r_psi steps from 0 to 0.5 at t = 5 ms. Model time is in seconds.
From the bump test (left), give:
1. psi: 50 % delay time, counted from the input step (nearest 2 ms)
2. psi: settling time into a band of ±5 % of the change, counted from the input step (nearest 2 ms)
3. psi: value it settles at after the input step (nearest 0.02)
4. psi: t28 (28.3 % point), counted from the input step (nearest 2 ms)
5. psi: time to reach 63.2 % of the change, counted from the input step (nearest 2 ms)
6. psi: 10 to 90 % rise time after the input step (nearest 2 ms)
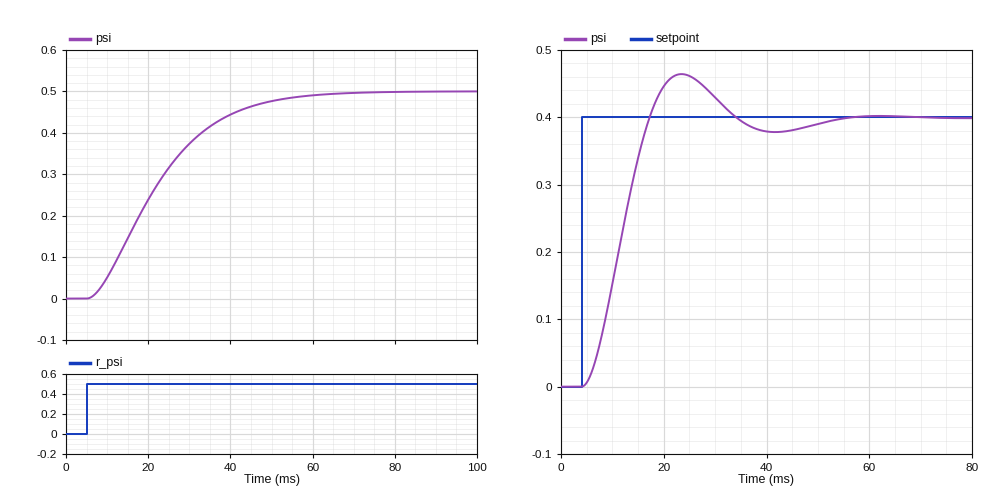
16 ms
44 ms
0.50
10 ms
20 ms
32 ms
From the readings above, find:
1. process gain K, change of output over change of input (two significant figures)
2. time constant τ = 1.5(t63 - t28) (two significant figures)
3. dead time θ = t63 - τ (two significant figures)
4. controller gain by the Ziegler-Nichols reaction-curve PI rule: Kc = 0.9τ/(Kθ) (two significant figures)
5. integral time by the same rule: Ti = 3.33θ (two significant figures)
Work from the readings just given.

1.0
15 ms
5.0 ms
2.7
17 ms
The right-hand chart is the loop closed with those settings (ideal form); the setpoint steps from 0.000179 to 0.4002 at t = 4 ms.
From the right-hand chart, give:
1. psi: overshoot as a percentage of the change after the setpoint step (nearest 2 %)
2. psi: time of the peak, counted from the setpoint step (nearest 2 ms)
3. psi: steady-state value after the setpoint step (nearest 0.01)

16 %
20 ms
0.40
